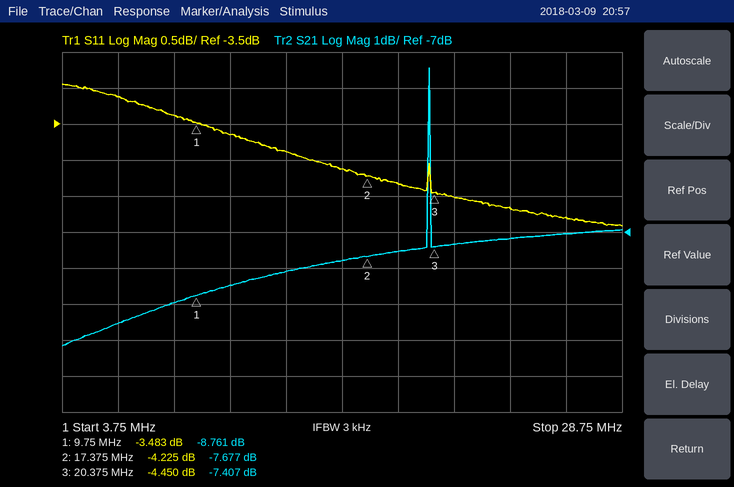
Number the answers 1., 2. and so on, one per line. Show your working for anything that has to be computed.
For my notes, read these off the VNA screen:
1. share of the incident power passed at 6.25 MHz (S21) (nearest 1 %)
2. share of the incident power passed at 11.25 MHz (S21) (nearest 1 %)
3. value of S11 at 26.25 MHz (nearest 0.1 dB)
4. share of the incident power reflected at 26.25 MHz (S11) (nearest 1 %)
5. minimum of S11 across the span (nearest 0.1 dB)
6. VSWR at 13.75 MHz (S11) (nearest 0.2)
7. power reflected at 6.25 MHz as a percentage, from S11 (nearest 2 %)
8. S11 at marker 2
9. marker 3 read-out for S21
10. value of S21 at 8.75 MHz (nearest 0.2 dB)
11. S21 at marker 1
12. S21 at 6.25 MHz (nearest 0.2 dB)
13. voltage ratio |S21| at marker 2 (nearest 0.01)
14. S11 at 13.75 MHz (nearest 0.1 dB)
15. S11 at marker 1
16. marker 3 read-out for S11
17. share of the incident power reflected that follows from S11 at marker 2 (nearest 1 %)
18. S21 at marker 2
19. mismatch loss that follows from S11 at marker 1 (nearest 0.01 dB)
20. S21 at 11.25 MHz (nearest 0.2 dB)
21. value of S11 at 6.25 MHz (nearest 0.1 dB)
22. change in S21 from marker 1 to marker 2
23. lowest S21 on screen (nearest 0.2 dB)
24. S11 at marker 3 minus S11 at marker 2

1. 10^(-9.6/10) ≈ 11 %
2. 10^(-8.4/10) ≈ 14 %
3. -4.8 dB
4. 10^(-4.8/10) ≈ 33 %
5. -4.9 dB
6. |Γ| = 10^(-3.9/20) = 0.6383; VSWR = (1 + 0.6383)/(1 − 0.6383) ≈ 4.53, so 4.6 to the nearest 0.2
7. 10^(-3.1/10) ≈ 49.0 %, so 48 % to the nearest 2 %
8. -4.225 dB
9. -7.407 dB
10. -9.0 dB
11. -8.761 dB
12. -9.6 dB
13. 10^(-7.677/20) ≈ 0.41
14. -3.9 dB
15. -3.483 dB
16. -4.450 dB
17. 10^(-4.225/10) ≈ 38 %
18. -7.677 dB
19. −10 log10(1 − 10^(-3.483/10)) ≈ 2.58 dB
20. -8.4 dB
21. -3.1 dB
22. -7.677 − (-8.761) = 1.084 dB
23. -10.2 dB
24. -4.45 − (-4.225) = -0.225 dB
